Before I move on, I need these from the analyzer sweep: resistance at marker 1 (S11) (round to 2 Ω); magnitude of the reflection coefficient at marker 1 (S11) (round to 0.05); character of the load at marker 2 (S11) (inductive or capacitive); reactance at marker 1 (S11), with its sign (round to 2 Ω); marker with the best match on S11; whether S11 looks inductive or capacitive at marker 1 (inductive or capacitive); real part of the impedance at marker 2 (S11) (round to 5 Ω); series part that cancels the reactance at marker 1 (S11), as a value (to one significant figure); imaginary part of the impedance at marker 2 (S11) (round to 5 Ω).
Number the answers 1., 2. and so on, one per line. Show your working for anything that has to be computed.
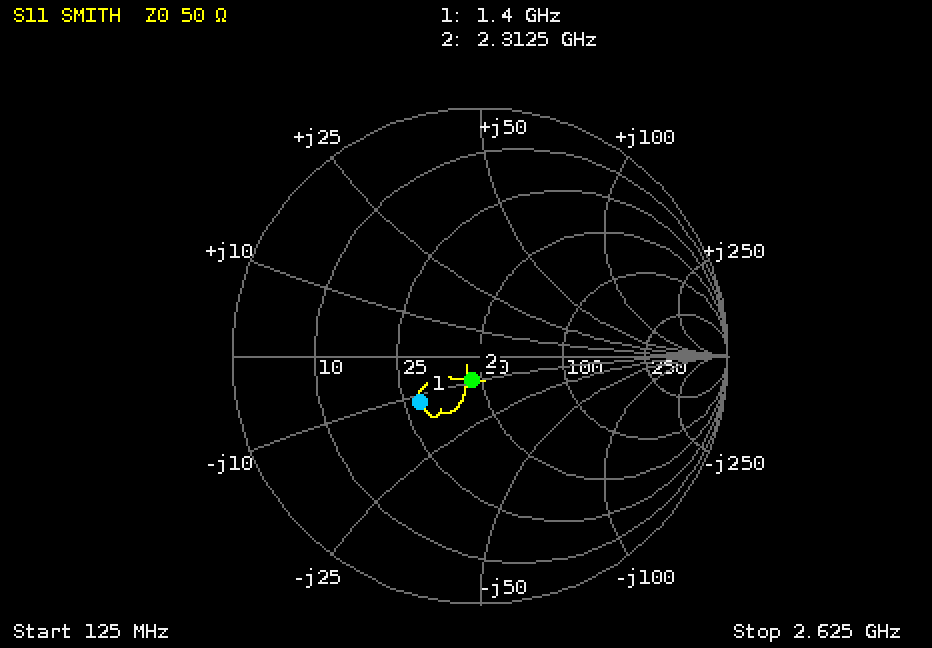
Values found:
1. 28 Ω
2. 0.30
3. capacitive
4. -12 Ω
5. marker 2
6. capacitive
7. 45 Ω
8. L = 12 Ω/(2π × 1.4 GHz) ≈ 1 nH
9. -10 Ω
